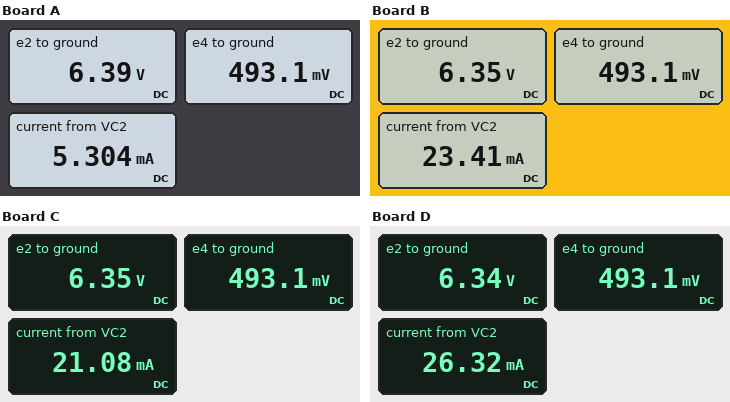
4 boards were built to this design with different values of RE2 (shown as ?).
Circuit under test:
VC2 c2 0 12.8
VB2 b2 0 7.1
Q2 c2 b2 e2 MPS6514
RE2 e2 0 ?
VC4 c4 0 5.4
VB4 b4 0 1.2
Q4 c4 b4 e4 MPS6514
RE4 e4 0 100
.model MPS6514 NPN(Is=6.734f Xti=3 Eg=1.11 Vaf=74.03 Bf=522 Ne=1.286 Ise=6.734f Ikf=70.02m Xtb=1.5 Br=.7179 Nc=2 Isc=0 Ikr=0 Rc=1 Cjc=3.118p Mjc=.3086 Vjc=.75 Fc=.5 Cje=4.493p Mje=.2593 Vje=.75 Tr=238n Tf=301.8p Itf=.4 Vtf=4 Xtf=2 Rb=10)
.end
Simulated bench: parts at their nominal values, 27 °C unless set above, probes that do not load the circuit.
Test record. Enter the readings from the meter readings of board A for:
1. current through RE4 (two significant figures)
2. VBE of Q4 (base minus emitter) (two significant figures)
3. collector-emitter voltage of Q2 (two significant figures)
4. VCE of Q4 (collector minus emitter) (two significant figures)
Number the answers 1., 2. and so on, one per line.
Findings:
1. 4.9 mA
2. 710 mV
3. 6.4 V
4. 4.9 V
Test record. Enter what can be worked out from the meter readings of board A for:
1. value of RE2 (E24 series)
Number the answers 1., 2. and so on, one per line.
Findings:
1. 1.2 kΩ
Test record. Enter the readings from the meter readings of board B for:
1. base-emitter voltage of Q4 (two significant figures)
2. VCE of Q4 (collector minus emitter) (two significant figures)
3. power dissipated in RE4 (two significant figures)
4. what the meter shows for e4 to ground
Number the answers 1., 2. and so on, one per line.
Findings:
1. 710 mV
2. 4.9 V
3. 2.4 mW
4. 493.1 mV
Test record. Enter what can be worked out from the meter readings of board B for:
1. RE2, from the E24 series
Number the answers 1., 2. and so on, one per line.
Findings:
1. 270 Ω
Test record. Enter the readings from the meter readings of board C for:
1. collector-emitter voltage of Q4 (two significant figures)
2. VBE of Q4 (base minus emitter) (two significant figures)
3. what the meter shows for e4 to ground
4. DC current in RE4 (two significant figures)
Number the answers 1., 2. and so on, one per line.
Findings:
1. 4.9 V
2. 710 mV
3. 493.1 mV
4. 4.9 mA
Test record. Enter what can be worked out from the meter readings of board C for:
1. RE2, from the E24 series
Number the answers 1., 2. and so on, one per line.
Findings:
1. 300 Ω
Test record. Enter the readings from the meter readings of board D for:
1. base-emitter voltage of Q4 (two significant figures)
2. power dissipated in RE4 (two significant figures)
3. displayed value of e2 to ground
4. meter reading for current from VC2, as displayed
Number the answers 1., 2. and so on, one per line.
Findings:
1. 710 mV
2. 2.4 mW
3. 6.34 V
4. 26.32 mA
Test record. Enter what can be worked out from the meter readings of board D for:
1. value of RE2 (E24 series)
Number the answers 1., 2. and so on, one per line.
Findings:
1. 240 Ω
